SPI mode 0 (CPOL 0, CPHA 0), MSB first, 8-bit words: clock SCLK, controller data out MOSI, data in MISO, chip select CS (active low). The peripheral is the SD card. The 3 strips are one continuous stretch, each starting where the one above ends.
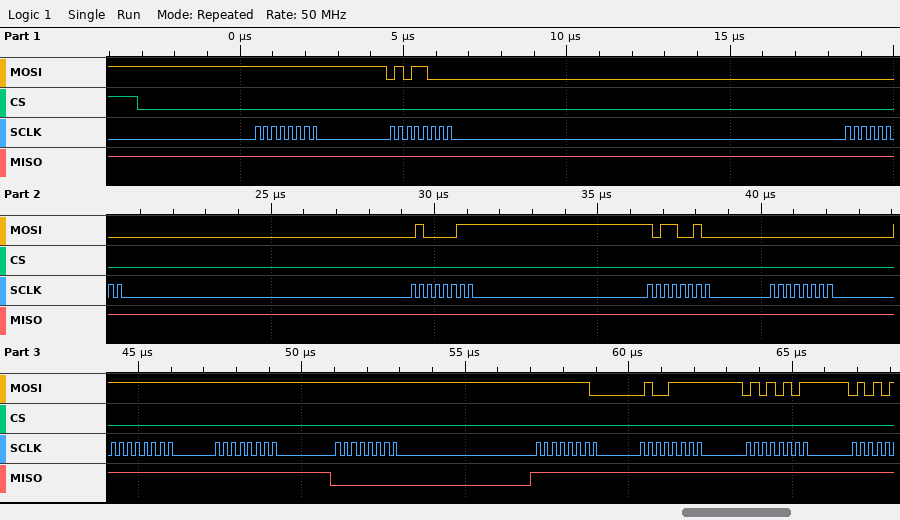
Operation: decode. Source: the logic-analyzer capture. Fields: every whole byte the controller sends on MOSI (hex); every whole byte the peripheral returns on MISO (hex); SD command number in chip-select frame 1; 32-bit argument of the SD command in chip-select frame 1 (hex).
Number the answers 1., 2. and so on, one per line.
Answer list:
1. FF 58 00 43 B2 00 FF FF FF FE 4F 55
2. FF FF FF FF FF FF FF FF 00 FF FF FF
3. CMD24
4. 0x0043B200
